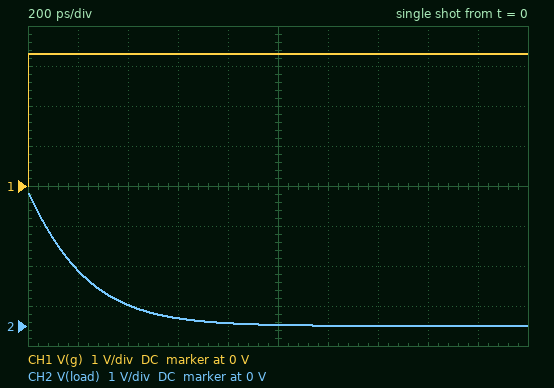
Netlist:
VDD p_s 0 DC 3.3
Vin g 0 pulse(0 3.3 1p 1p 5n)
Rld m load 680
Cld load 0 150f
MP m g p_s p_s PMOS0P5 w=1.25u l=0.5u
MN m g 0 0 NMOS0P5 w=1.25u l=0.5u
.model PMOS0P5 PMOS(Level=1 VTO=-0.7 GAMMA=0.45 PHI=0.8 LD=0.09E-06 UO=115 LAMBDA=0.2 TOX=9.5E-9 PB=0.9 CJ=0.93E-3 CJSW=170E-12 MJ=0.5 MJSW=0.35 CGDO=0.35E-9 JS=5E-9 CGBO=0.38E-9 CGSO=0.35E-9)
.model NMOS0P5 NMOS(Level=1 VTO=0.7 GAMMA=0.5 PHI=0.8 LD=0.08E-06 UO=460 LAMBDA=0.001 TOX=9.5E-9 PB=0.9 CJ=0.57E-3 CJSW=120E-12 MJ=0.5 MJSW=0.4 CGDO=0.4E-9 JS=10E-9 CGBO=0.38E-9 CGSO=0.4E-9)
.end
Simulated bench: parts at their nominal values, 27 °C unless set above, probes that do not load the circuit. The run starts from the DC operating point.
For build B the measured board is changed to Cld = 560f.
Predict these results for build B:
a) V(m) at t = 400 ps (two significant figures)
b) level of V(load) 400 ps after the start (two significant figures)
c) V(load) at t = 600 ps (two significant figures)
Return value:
1.1 V
2.1 V
1.6 V
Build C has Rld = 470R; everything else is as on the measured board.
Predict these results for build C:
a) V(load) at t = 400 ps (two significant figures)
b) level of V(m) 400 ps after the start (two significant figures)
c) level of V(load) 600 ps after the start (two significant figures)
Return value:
390 mV
230 mV
120 mV
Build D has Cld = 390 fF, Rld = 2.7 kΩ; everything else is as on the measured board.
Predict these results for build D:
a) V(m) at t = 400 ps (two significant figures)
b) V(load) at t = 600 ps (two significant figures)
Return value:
500 mV
2.1 V
